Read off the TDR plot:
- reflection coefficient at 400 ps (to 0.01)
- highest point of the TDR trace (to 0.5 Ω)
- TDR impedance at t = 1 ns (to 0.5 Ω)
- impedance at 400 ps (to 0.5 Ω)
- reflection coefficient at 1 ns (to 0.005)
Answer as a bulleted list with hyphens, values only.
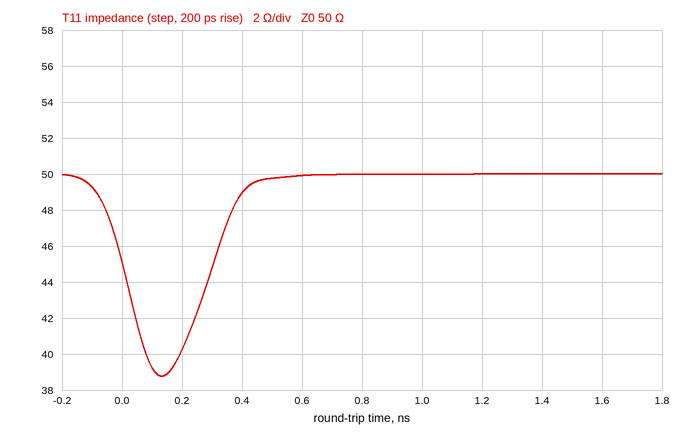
- -0.01
- 50.0 Ω
- 50.0 Ω
- 49.0 Ω
- 0.000
